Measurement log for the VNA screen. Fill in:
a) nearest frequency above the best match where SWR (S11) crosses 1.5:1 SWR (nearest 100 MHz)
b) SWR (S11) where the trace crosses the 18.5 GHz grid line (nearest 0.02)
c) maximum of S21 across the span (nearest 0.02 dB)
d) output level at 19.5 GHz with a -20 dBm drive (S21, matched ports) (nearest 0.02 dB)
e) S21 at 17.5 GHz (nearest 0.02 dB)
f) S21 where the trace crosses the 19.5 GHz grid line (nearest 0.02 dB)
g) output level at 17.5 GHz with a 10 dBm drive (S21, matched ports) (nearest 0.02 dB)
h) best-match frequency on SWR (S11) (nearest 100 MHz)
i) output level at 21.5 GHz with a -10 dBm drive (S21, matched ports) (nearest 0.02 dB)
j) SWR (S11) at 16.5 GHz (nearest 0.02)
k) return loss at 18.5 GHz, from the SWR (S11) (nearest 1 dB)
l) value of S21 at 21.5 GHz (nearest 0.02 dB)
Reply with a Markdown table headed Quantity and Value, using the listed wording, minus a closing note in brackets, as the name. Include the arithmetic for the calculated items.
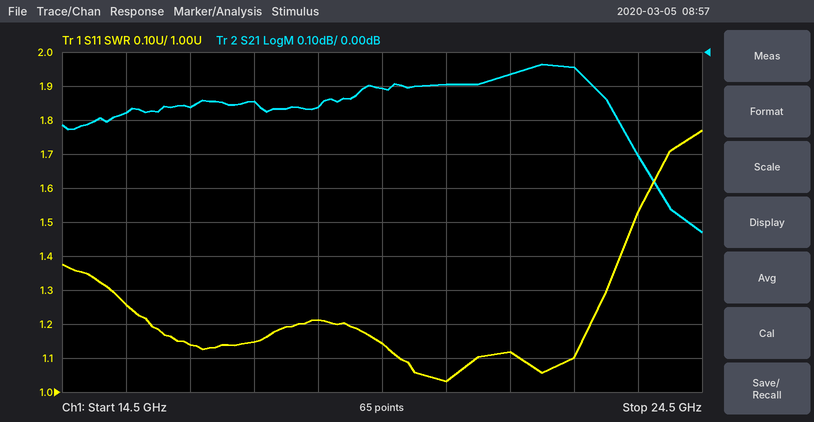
| Quantity | Value |
|---|---|
| nearest frequency above the best match where SWR (S11) crosses 1.5:1 SWR | 23.4 GHz |
| SWR (S11) where the trace crosses the 18.5 GHz grid line | 1.22 |
| maximum of S21 across the span | -0.04 dB |
| output level at 19.5 GHz with a -20 dBm drive (S21, matched ports) | -20 dBm + (-0.10 dB) = -20.10 dBm |
| S21 at 17.5 GHz | -0.14 dB |
| S21 where the trace crosses the 19.5 GHz grid line | -0.10 dB |
| output level at 17.5 GHz with a 10 dBm drive (S21, matched ports) | 10 dBm + (-0.14 dB) = 9.86 dBm |
| best-match frequency on SWR (S11) | 20.5 GHz |
| output level at 21.5 GHz with a -10 dBm drive (S21, matched ports) | -10 dBm + (-0.06 dB) = -10.06 dBm |
| SWR (S11) at 16.5 GHz | 1.14 |
| return loss at 18.5 GHz, from the SWR (S11) | −20 log10((1.22 − 1)/(1.22 + 1)) ≈ 20 dB |
| value of S21 at 21.5 GHz | -0.06 dB |
